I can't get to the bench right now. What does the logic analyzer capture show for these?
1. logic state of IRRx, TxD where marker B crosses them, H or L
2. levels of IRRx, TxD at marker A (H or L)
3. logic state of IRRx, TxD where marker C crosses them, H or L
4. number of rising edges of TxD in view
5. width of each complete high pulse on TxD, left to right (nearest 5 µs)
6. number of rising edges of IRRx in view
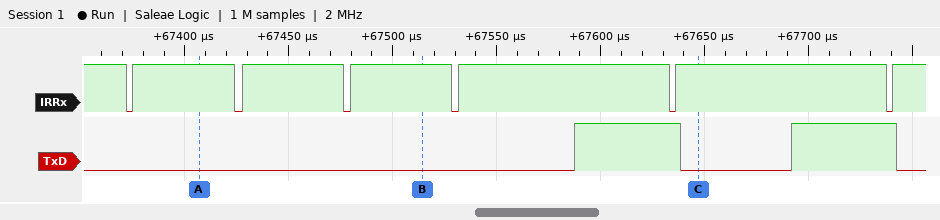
IRRx=H, TxD=L
IRRx=H, TxD=L
IRRx=H, TxD=L
2
50 µs, 50 µs
6
